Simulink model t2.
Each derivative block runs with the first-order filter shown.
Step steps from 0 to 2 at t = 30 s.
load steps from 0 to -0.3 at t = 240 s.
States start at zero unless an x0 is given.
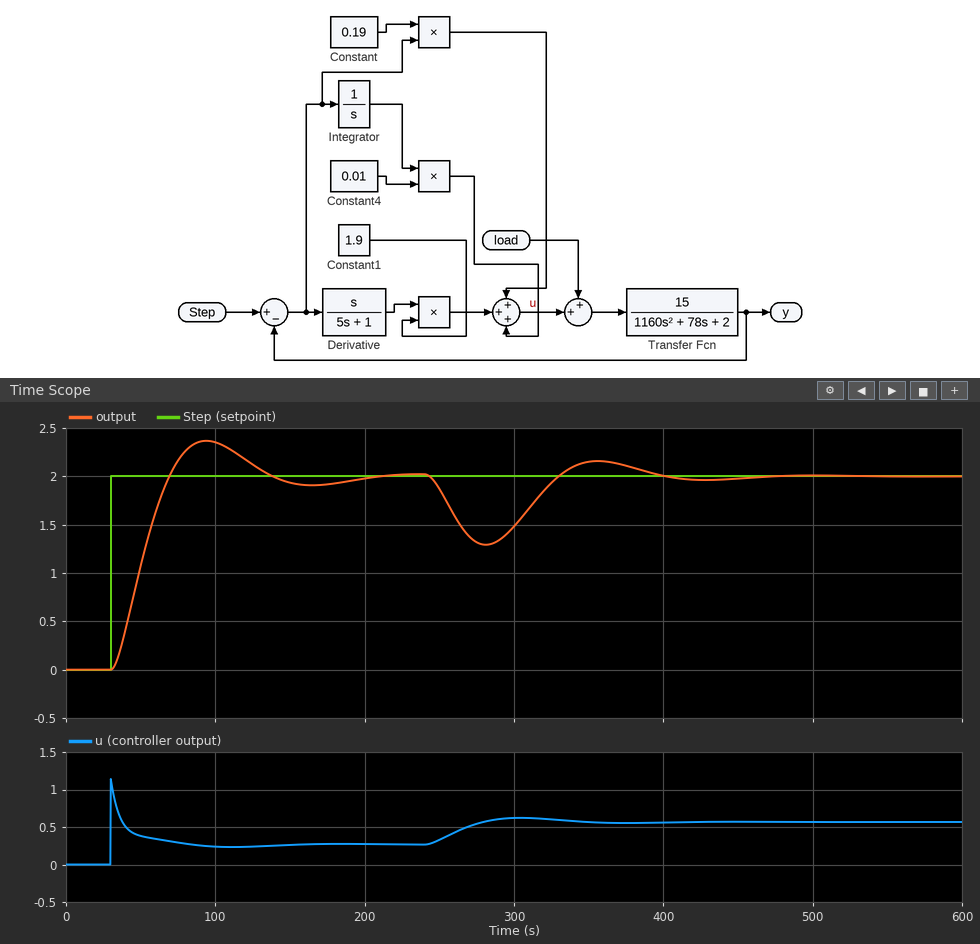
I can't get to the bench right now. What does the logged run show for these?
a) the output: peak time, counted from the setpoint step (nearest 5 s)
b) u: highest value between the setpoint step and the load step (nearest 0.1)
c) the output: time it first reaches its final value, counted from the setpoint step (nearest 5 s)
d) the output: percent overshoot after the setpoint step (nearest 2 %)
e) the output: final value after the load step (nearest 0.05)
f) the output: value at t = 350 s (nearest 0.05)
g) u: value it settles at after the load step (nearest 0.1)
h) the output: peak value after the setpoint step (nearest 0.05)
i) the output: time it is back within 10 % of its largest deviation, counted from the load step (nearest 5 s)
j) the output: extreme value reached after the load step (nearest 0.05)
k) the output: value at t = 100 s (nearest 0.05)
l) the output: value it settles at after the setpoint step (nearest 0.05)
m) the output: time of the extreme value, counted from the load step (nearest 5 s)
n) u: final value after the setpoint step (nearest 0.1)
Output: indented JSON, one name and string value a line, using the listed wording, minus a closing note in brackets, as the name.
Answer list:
{
  "the output: peak time, counted from the setpoint step": "65 s",
  "u: highest value between the setpoint step and the load step": "1.1",
  "the output: time it first reaches its final value, counted from the setpoint step": "40 s",
  "the output: percent overshoot after the setpoint step": "18 %",
  "the output: final value after the load step": "2.00",
  "the output: value at t = 350 s": "2.15",
  "u: value it settles at after the load step": "0.6",
  "the output: peak value after the setpoint step": "2.35",
  "the output: time it is back within 10 % of its largest deviation, counted from the load step": "145 s",
  "the output: extreme value reached after the load step": "1.30",
  "the output: value at t = 100 s": "2.35",
  "the output: value it settles at after the setpoint step": "2.00",
  "the output: time of the extreme value, counted from the load step": "40 s",
  "u: final value after the setpoint step": "0.3"
}
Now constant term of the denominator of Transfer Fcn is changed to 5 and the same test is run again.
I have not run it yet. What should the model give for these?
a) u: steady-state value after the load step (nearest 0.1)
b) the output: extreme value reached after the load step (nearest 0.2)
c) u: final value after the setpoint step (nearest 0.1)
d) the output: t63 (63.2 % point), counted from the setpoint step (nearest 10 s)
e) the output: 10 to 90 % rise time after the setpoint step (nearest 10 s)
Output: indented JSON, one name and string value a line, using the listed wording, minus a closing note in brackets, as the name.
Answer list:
{
  "u: steady-state value after the load step": "1.0",
  "the output: extreme value reached after the load step": "1.4",
  "u: final value after the setpoint step": "0.7",
  "the output: t63 (63.2 % point), counted from the setpoint step": "30 s",
  "the output: 10 to 90 % rise time after the setpoint step": "80 s"
}
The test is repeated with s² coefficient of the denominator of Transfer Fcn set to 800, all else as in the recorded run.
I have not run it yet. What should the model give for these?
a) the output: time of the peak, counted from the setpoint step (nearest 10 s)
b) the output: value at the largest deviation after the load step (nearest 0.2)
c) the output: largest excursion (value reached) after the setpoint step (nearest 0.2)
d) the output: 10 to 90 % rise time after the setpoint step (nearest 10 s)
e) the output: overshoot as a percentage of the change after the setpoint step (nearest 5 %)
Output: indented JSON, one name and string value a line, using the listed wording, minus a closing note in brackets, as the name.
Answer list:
{
  "the output: time of the peak, counted from the setpoint step": "70 s",
  "the output: value at the largest deviation after the load step": "1.4",
  "the output: largest excursion (value reached) after the setpoint step": "2.2",
  "the output: 10 to 90 % rise time after the setpoint step": "30 s",
  "the output: overshoot as a percentage of the change after the setpoint step": "10 %"
}
